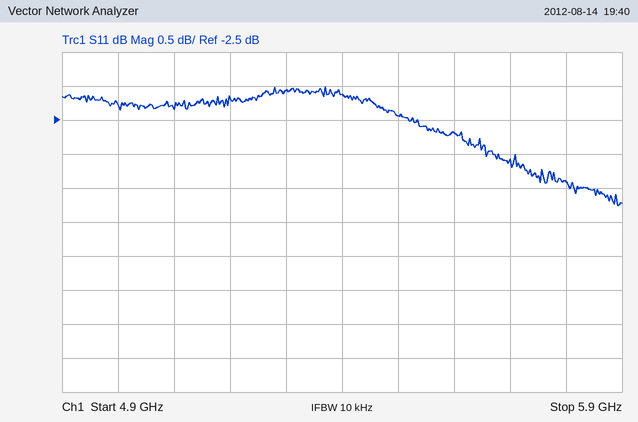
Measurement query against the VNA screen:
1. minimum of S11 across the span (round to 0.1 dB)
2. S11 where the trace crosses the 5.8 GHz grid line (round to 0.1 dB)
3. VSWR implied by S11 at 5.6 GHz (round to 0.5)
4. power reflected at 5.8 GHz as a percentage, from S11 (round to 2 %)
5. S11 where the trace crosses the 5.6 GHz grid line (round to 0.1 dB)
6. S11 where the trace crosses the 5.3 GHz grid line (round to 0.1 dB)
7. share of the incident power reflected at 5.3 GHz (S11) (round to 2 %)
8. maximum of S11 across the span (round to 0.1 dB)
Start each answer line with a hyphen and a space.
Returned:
- -3.8 dB
- -3.4 dB
- 6.5
- 46 %
- -2.7 dB
- -2.1 dB
- 62 %
- -2.0 dB
